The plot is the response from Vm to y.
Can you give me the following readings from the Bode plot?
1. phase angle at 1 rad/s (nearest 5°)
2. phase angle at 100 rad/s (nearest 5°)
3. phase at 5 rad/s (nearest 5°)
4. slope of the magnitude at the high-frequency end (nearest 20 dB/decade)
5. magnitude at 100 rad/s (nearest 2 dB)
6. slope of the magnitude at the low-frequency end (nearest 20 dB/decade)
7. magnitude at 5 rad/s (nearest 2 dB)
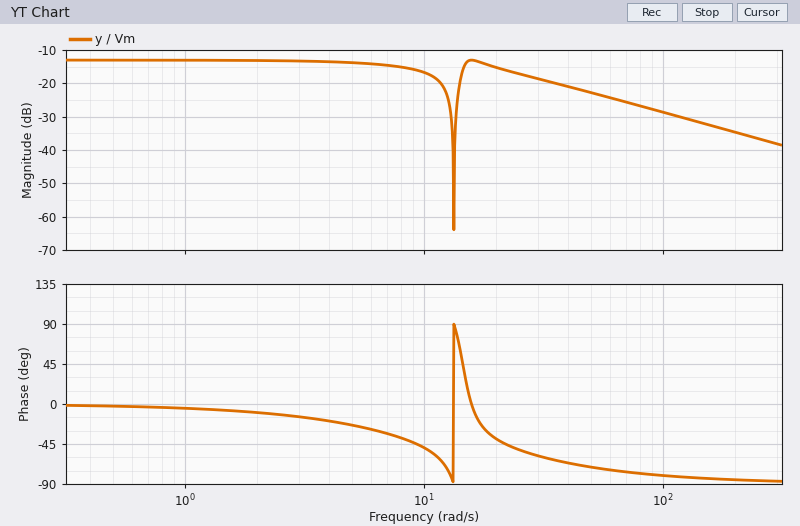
-5°
-80°
-25°
-20 dB/decade
-28 dB
0 dB/decade
-14 dB
